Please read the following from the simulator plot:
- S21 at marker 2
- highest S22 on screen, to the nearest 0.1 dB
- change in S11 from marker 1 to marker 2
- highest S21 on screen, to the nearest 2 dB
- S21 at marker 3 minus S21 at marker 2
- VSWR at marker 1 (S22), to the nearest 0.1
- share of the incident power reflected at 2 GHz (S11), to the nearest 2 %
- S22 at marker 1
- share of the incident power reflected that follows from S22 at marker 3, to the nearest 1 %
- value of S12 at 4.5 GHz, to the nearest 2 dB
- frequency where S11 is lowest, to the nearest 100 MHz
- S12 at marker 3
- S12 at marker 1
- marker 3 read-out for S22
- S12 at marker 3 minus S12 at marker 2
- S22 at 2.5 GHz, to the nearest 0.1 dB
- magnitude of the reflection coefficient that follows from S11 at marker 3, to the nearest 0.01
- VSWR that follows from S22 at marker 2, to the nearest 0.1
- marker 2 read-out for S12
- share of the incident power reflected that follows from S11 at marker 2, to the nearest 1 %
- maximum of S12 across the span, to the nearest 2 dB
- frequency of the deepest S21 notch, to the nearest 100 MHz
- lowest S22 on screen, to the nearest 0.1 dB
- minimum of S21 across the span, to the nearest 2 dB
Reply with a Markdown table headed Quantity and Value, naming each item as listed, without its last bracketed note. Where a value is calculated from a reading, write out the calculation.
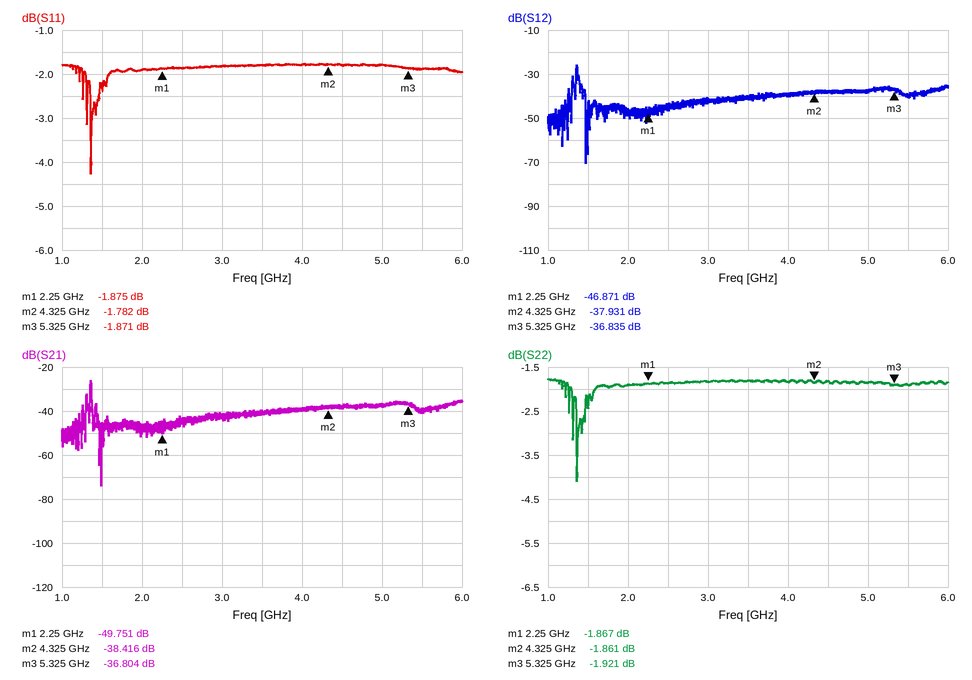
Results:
| Quantity | Value |
|---|---|
| S21 at marker 2 | -38.416 dB |
| highest S22 on screen, to the nearest 0.1 dB | -1.8 dB |
| change in S11 from marker 1 to marker 2 | -1.782 − (-1.875) = 0.093 dB |
| highest S21 on screen, to the nearest 2 dB | -26 dB |
| S21 at marker 3 minus S21 at marker 2 | -36.804 − (-38.416) = 1.612 dB |
| VSWR at marker 1 (S22), to the nearest 0.1 | (1 + 0.8066)/(1 − 0.8066) ≈ 9.3 |
| share of the incident power reflected at 2 GHz (S11), to the nearest 2 % | 10^(-1.9/10) ≈ 64.6 %, so 64 % to the nearest 2 % |
| S22 at marker 1 | -1.867 dB |
| share of the incident power reflected that follows from S22 at marker 3, to the nearest 1 % | 10^(-1.921/10) ≈ 64 % |
| value of S12 at 4.5 GHz, to the nearest 2 dB | -38 dB |
| frequency where S11 is lowest, to the nearest 100 MHz | 1.4 GHz |
| S12 at marker 3 | -36.835 dB |
| S12 at marker 1 | -46.871 dB |
| marker 3 read-out for S22 | -1.921 dB |
| S12 at marker 3 minus S12 at marker 2 | -36.835 − (-37.931) = 1.096 dB |
| S22 at 2.5 GHz, to the nearest 0.1 dB | -1.9 dB |
| magnitude of the reflection coefficient that follows from S11 at marker 3, to the nearest 0.01 | 10^(-1.871/20) ≈ 0.81 |
| VSWR that follows from S22 at marker 2, to the nearest 0.1 | (1 + 0.8071)/(1 − 0.8071) ≈ 9.4 |
| marker 2 read-out for S12 | -37.931 dB |
| share of the incident power reflected that follows from S11 at marker 2, to the nearest 1 % | 10^(-1.782/10) ≈ 66 % |
| maximum of S12 across the span, to the nearest 2 dB | -26 dB |
| frequency of the deepest S21 notch, to the nearest 100 MHz | 1.5 GHz |
| lowest S22 on screen, to the nearest 0.1 dB | -4.1 dB |
| minimum of S21 across the span, to the nearest 2 dB | -74 dB |
